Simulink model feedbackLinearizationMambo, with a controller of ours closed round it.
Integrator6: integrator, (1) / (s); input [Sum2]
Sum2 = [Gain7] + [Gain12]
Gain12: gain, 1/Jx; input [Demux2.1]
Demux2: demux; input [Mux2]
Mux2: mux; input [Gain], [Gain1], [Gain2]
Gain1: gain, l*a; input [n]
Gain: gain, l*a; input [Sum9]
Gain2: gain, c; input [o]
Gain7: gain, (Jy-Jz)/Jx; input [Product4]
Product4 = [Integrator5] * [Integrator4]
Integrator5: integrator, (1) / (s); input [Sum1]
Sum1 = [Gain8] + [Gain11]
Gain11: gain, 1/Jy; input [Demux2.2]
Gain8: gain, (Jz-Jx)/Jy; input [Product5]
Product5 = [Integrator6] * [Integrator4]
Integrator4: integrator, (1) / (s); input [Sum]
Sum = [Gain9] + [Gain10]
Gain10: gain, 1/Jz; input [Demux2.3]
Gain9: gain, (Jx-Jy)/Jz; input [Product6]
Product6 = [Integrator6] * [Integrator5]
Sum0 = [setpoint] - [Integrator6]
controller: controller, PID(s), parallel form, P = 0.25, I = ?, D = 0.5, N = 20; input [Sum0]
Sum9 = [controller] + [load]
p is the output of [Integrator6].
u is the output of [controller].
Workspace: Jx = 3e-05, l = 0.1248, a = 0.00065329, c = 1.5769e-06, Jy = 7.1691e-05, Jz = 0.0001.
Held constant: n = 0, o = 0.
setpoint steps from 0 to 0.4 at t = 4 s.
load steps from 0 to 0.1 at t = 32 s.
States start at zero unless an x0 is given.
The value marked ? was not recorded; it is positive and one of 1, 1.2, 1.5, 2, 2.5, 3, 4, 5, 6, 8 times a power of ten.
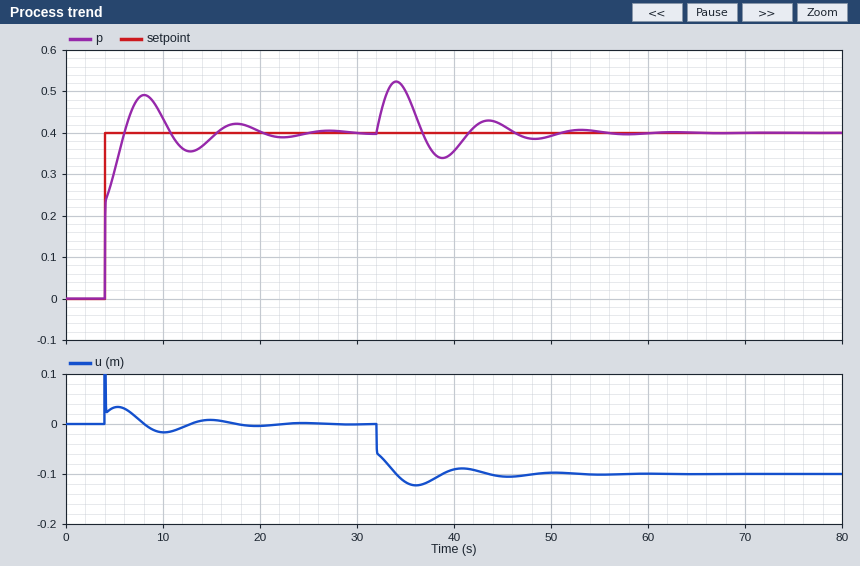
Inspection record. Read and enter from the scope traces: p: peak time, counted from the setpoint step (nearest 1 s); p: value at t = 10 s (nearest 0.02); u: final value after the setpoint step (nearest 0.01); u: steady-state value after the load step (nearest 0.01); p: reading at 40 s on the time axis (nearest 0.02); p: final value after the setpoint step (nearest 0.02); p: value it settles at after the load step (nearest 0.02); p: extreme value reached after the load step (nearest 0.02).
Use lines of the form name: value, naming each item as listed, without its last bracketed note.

p: peak time, counted from the setpoint step: 4 s
p: value at t = 10 s: 0.44
u: final value after the setpoint step: 0.00
u: steady-state value after the load step: -0.10
p: reading at 40 s on the time axis: 0.36
p: final value after the setpoint step: 0.40
p: value it settles at after the load step: 0.40
p: extreme value reached after the load step: 0.52
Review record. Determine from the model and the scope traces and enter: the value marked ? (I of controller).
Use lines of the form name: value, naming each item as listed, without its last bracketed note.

the value marked ?: 0.4
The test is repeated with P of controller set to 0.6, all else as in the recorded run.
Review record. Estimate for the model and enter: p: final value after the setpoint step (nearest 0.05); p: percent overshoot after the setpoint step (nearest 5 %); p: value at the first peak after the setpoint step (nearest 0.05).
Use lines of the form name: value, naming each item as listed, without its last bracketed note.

p: final value after the setpoint step: 0.40
p: percent overshoot after the setpoint step: 10 %
p: value at the first peak after the setpoint step: 0.45
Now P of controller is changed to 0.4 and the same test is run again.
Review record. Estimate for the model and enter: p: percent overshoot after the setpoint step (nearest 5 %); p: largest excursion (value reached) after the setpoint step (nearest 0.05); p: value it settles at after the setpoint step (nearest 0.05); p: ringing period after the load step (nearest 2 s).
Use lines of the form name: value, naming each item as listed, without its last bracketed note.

p: percent overshoot after the setpoint step: 15 %
p: largest excursion (value reached) after the setpoint step: 0.45
p: value it settles at after the setpoint step: 0.40
p: ringing period after the load step: 10 s
